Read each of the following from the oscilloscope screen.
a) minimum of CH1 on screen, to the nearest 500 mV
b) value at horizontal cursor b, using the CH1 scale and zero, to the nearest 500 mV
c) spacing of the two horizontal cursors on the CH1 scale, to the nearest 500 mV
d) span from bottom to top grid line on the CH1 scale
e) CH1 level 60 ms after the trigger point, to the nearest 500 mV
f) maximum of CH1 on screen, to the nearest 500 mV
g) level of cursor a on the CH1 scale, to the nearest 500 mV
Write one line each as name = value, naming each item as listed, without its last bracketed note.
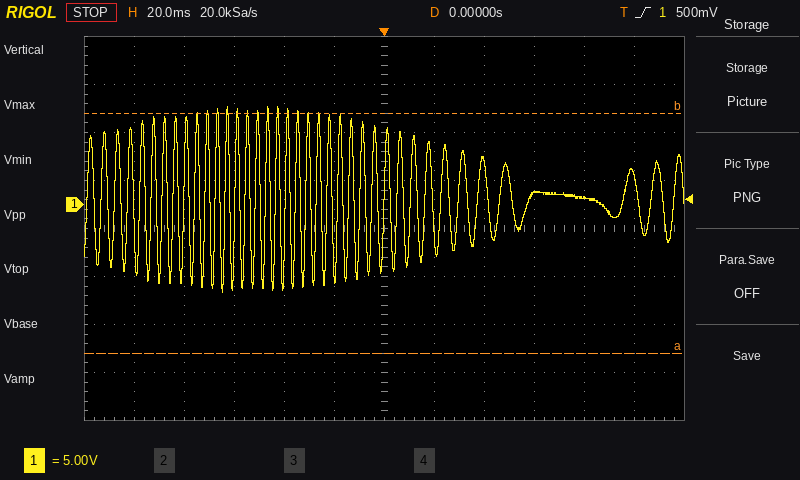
minimum of CH1 on screen, to the nearest 500 mV = -9.0 V
value at horizontal cursor b, using the CH1 scale and zero, to the nearest 500 mV = 9.5 V
spacing of the two horizontal cursors on the CH1 scale, to the nearest 500 mV = 25.0 V
span from bottom to top grid line on the CH1 scale = 40 V
CH1 level 60 ms after the trigger point, to the nearest 500 mV = 1.0 V
maximum of CH1 on screen, to the nearest 500 mV = 10.0 V
level of cursor a on the CH1 scale, to the nearest 500 mV = -15.5 V
